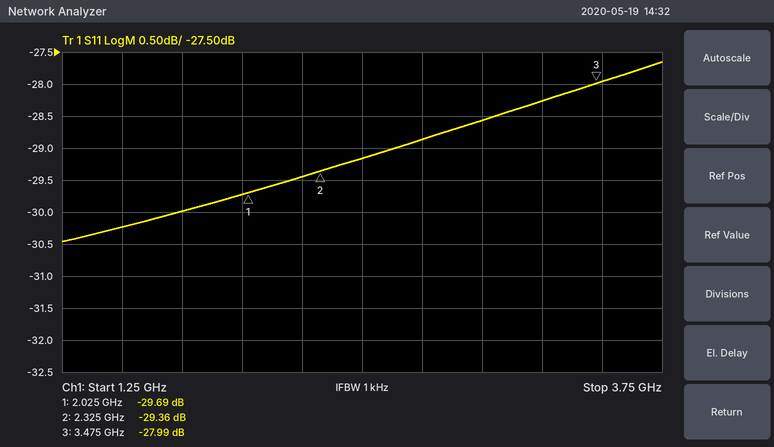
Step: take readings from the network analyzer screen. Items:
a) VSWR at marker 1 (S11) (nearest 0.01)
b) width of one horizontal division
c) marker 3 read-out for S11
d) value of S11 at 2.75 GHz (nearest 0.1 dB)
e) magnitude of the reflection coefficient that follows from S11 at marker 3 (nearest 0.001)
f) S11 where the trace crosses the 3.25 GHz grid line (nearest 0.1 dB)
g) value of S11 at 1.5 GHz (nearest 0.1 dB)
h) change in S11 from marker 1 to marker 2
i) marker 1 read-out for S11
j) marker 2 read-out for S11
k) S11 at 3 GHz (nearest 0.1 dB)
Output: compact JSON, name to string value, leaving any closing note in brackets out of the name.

{"VSWR at marker 1 (S11)": "1.07", "width of one horizontal division": "250 MHz", "marker 3 read-out for S11": "-27.99 dB", "value of S11 at 2.75 GHz": "-28.9 dB", "magnitude of the reflection coefficient that follows from S11 at marker 3": "0.040", "S11 where the trace crosses the 3.25 GHz grid line": "-28.3 dB", "value of S11 at 1.5 GHz": "-30.2 dB", "change in S11 from marker 1 to marker 2": "0.33 dB", "marker 1 read-out for S11": "-29.69 dB", "marker 2 read-out for S11": "-29.36 dB", "S11 at 3 GHz": "-28.6 dB"}
